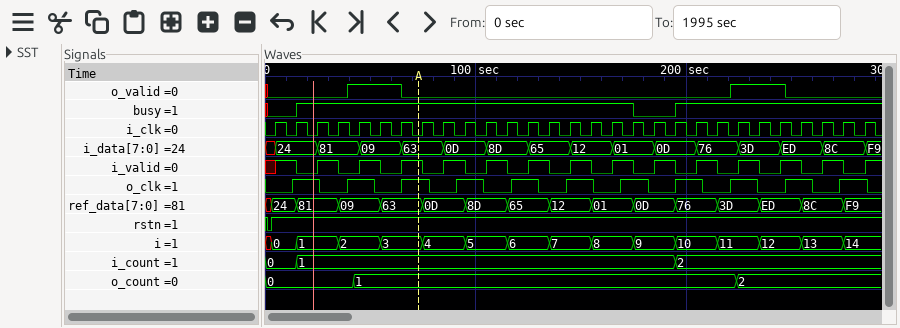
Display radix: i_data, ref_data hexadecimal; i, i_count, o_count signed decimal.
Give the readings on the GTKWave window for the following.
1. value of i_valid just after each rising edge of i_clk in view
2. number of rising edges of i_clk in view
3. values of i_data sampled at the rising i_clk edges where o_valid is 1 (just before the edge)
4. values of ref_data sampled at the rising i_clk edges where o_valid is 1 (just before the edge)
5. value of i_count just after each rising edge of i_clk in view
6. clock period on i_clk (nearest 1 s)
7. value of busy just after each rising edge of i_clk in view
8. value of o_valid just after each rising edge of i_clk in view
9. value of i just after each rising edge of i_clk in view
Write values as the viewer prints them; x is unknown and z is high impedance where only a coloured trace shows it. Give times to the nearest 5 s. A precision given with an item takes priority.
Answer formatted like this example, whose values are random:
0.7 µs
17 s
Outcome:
1 0 1 0 1 0 1 0 1 0 1 0 1 0 1 0 1 0 1 0 1 0 1 0 1 0 1 0 1
29
81, 09, 09, 76, 3D, 3D
09, 09, 63, 3D, 3D, ED
0, 1, 1, 1, 1, 1, 1, 1, 1, 1, 1, 1, 1, 1, 1, 1, 1, 1, 1, 2, 2, 2, 2, 2, 2, 2, 2, 2, 2
10 s
0 1 1 1 1 1 1 1 1 1 1 1 1 1 1 1 1 0 0 1 1 1 1 1 1 1 1 1 1
0 0 0 0 1 1 0 0 0 0 0 0 0 0 0 0 0 0 0 0 0 0 1 1 1 0 0 0 0
0, 1, 1, 2, 2, 3, 3, 4, 4, 5, 5, 6, 6, 7, 7, 8, 8, 9, 9, 10, 10, 11, 11, 12, 12, 13, 13, 14, 14
